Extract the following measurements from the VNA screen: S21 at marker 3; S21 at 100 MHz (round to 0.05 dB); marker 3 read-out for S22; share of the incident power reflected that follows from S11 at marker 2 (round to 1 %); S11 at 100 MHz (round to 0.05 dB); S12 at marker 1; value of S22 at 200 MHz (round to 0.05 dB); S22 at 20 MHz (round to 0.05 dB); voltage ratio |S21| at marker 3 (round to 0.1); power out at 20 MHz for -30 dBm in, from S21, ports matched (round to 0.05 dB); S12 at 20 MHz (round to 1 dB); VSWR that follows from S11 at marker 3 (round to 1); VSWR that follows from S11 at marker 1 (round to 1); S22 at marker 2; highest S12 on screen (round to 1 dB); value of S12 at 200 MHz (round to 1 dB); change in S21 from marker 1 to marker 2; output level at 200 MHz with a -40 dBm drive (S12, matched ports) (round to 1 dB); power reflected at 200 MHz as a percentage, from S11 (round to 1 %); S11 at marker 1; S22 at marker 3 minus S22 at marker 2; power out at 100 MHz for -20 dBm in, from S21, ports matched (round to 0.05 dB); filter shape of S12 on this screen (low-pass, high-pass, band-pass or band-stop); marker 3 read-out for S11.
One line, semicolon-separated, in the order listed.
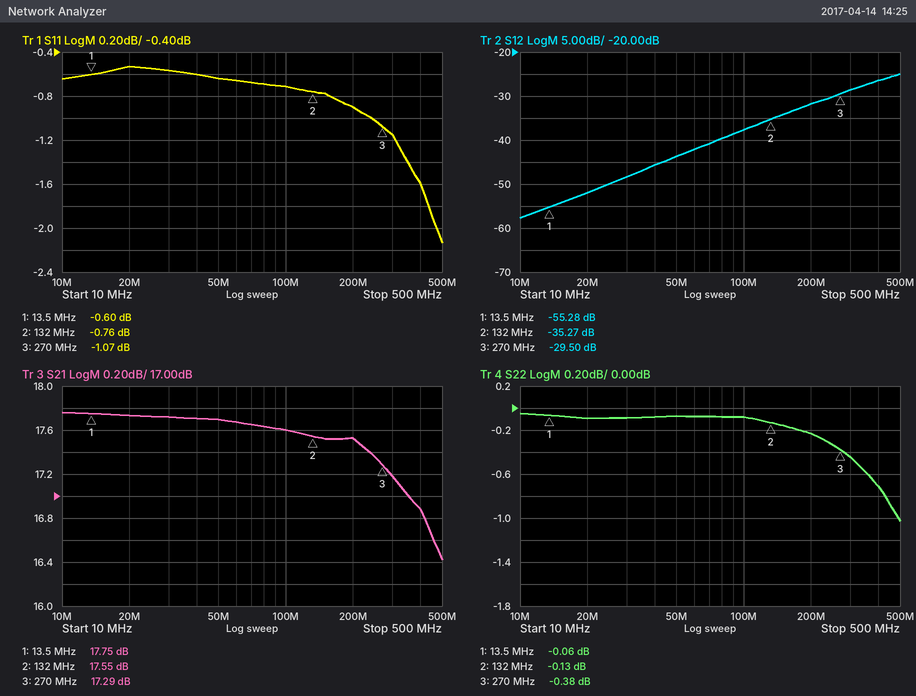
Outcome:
17.29 dB; 17.60 dB; -0.38 dB; 84 %; -0.70 dB; -55.28 dB; -0.25 dB; -0.10 dB; 7.3; -12.25 dBm; -52 dB; 16; 29; -0.13 dB; -25 dB; -32 dB; -0.20 dB; -72 dBm; 81 %; -0.60 dB; -0.25 dB; -2.40 dBm; high-pass; -1.07 dB
